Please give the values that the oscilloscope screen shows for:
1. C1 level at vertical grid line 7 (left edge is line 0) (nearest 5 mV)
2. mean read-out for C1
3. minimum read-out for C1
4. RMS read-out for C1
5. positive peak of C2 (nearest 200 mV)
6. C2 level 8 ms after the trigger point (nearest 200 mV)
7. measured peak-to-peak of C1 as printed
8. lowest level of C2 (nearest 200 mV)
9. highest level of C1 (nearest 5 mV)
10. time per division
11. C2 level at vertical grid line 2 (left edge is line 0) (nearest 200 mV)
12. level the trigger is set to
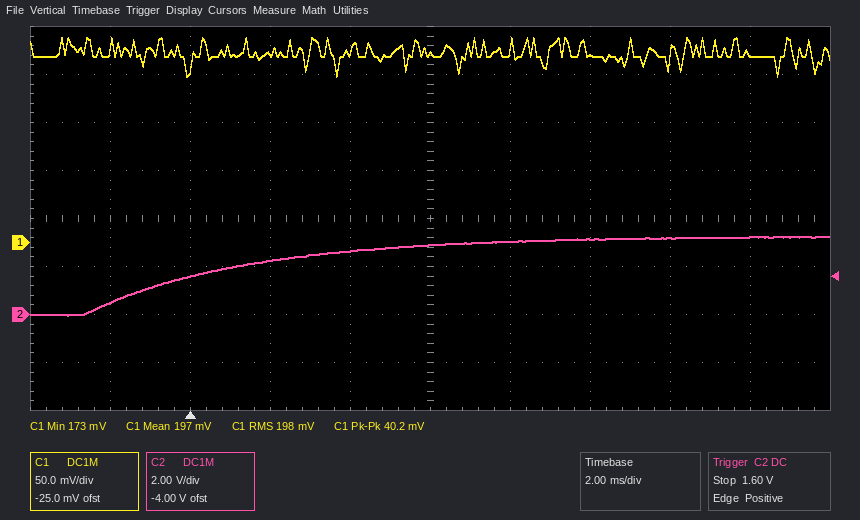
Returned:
195 mV
197 mV
173 mV
198 mV
3.2 V
3.0 V
40.2 mV
0.0 V
215 mV
2 ms
1.6 V
1.60 V
